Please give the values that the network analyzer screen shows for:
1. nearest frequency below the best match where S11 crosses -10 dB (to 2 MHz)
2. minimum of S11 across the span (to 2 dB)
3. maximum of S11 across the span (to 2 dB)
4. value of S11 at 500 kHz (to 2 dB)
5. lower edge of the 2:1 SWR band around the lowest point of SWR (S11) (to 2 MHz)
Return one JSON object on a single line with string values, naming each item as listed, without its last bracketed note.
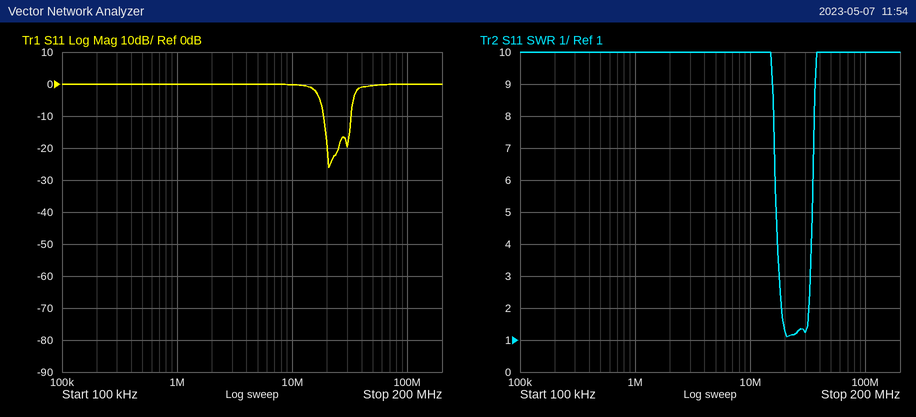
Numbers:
{"nearest frequency below the best match where S11 crosses -10 dB": "18 MHz", "minimum of S11 across the span": "-26 dB", "maximum of S11 across the span": "0 dB", "value of S11 at 500 kHz": "0 dB", "lower edge of the 2:1 SWR band around the lowest point of SWR (S11)": "18 MHz"}
